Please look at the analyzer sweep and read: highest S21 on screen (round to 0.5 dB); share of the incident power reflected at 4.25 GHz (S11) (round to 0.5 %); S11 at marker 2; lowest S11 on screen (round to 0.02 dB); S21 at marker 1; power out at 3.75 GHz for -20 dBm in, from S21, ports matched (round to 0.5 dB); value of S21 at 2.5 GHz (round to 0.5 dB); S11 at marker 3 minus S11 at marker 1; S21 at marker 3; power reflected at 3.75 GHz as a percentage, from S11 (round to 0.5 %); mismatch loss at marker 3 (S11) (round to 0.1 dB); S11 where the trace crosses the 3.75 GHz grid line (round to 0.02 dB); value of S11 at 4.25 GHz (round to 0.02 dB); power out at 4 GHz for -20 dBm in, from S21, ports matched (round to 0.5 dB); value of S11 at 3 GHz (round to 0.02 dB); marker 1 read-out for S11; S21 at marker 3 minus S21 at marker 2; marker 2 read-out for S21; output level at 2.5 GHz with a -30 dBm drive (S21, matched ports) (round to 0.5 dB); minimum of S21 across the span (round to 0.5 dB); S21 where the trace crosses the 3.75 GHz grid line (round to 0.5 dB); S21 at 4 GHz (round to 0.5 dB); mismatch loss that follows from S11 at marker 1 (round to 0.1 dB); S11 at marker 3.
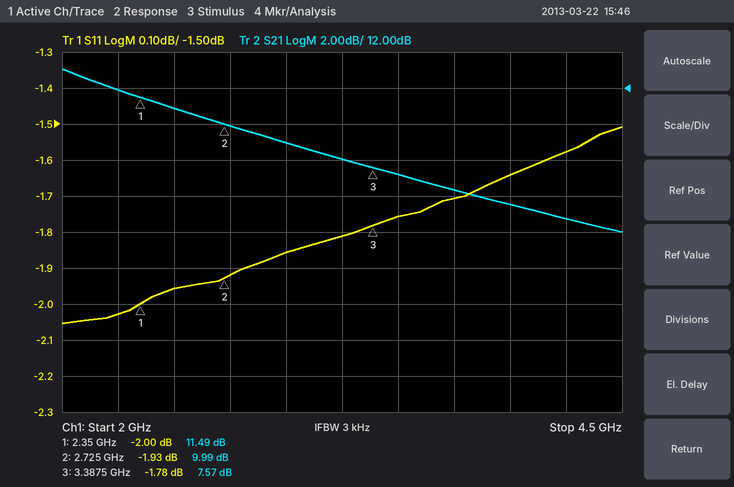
13.0 dB
69.5 %
-1.93 dB
-2.06 dB
11.49 dB
-13.5 dBm
11.0 dB
0.22 dB
7.57 dB
67.5 %
4.7 dB
-1.70 dB
-1.58 dB
-14.5 dBm
-1.86 dB
-2.00 dB
-2.42 dB
9.99 dB
-19.0 dBm
4.0 dB
6.5 dB
5.5 dB
4.3 dB
-1.78 dB
